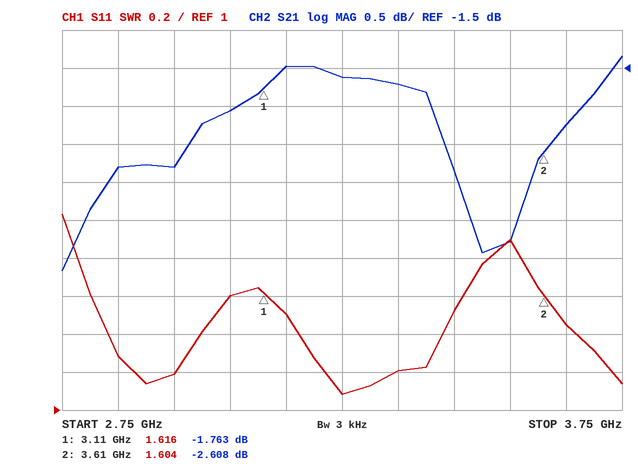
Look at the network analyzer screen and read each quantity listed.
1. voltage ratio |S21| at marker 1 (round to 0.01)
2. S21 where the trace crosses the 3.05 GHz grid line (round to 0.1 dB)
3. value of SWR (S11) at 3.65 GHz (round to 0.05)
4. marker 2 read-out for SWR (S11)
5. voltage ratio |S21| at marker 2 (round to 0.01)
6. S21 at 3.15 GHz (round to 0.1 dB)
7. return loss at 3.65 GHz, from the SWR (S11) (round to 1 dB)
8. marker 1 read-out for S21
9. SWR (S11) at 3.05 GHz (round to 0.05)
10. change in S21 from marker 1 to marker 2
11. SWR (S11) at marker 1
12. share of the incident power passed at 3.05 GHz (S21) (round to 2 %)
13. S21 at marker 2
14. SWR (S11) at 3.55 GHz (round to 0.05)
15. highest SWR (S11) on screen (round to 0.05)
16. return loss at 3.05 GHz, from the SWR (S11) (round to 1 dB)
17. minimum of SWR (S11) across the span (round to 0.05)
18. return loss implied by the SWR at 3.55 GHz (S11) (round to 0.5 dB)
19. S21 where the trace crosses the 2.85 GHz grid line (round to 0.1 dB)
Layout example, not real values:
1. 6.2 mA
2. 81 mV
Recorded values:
1. 0.82
2. -2.1 dB
3. 1.45
4. 1.604
5. 0.74
6. -1.5 dB
7. 15 dB
8. -1.763 dB
9. 1.60
10. -0.845 dB
11. 1.616
12. 62 %
13. -2.608 dB
14. 1.90
15. 2.05
16. 13 dB
17. 1.10
18. 10.0 dB
19. -2.8 dB
